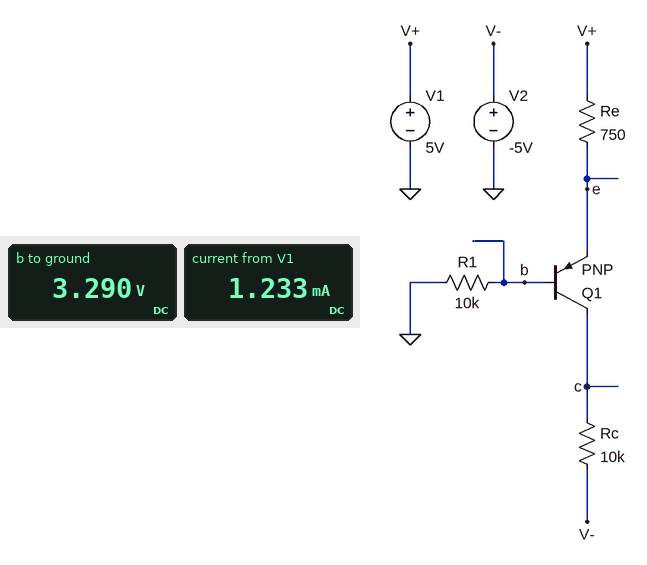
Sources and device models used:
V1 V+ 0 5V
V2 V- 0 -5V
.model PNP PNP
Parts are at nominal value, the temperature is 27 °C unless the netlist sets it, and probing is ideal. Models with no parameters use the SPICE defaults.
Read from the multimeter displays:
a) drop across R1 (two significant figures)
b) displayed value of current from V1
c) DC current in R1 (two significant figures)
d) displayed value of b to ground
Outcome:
3.3 V
1.233 mA
330 µA
3.290 V
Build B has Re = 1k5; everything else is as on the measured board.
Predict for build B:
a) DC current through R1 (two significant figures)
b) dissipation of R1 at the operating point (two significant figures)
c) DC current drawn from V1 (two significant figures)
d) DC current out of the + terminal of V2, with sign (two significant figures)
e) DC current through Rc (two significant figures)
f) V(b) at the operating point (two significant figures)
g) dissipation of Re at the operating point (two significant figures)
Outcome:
260 µA
670 µW
1.1 mA
-830 µA
830 µA
2.6 V
1.8 mW
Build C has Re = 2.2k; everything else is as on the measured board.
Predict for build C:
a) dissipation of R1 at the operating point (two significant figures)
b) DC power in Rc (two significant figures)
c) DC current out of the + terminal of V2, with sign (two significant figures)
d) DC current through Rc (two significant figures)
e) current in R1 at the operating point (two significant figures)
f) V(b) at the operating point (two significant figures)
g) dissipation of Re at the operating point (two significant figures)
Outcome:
420 µW
6.1 mW
-780 µA
780 µA
210 µA
2.1 V
2.1 mW
